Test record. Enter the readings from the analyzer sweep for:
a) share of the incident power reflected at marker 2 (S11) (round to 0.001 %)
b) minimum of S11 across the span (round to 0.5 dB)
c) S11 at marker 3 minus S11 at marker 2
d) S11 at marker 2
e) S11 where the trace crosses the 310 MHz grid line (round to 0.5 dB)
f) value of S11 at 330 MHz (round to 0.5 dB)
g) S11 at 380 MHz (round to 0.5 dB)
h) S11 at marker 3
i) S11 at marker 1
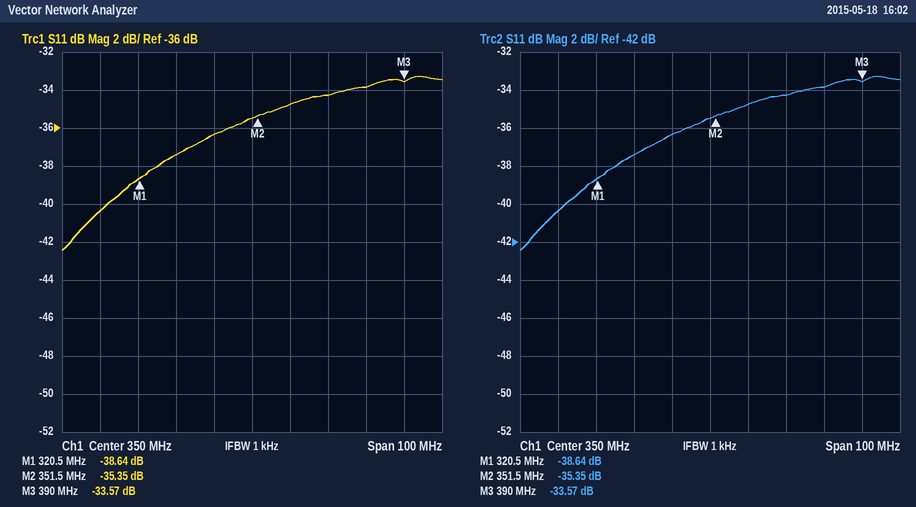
0.029 %
-42.5 dB
1.78 dB
-35.35 dB
-40.5 dB
-37.5 dB
-34.0 dB
-33.57 dB
-38.64 dB
